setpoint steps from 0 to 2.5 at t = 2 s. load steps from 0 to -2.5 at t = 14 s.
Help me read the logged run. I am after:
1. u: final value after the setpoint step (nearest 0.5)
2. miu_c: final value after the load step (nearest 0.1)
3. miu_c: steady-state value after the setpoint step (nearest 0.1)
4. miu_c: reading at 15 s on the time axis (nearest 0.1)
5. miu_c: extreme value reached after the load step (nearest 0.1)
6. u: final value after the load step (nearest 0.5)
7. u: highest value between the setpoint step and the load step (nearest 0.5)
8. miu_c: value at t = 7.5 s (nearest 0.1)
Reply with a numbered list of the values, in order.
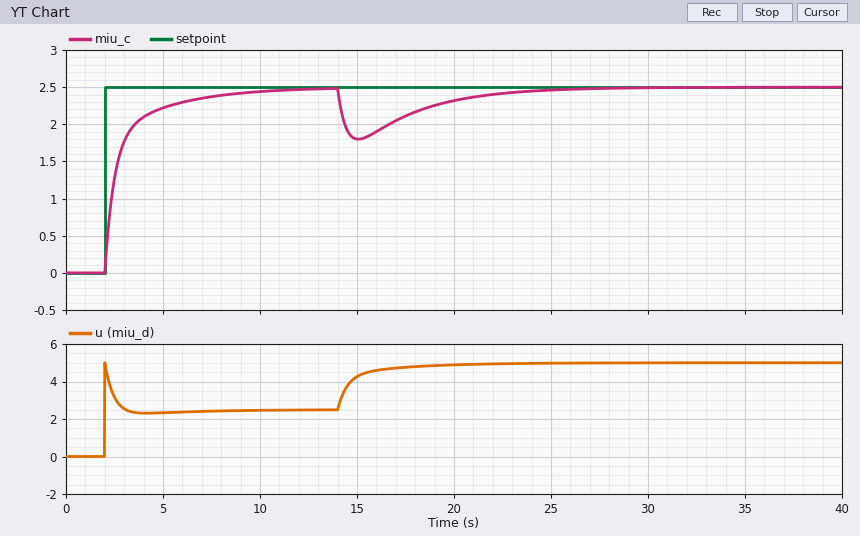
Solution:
1. 2.5
2. 2.5
3. 2.5
4. 1.8
5. 1.8
6. 5.0
7. 5.0
8. 2.4
